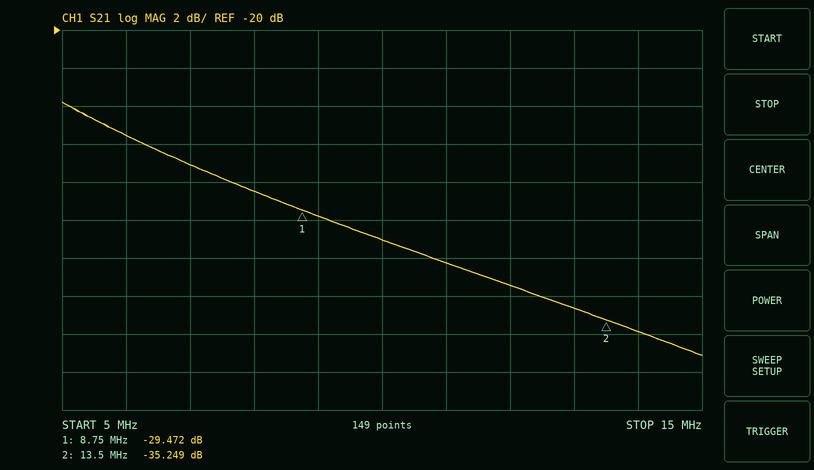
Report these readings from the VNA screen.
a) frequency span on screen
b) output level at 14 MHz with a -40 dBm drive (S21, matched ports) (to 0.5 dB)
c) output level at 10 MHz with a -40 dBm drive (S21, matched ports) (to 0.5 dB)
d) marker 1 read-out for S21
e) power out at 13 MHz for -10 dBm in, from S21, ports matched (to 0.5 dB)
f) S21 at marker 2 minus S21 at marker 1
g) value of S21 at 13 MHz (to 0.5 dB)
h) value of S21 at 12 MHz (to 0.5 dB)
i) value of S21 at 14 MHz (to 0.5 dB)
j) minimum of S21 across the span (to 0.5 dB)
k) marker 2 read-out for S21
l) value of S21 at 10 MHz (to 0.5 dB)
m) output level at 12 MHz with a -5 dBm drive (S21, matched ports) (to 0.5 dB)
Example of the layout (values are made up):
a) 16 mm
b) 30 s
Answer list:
a) 10 MHz
b) -76.0 dBm
c) -71.0 dBm
d) -29.472 dB
e) -44.5 dBm
f) -5.777 dB
g) -34.5 dB
h) -33.5 dB
i) -36.0 dB
j) -37.0 dB
k) -35.249 dB
l) -31.0 dB
m) -38.5 dBm
